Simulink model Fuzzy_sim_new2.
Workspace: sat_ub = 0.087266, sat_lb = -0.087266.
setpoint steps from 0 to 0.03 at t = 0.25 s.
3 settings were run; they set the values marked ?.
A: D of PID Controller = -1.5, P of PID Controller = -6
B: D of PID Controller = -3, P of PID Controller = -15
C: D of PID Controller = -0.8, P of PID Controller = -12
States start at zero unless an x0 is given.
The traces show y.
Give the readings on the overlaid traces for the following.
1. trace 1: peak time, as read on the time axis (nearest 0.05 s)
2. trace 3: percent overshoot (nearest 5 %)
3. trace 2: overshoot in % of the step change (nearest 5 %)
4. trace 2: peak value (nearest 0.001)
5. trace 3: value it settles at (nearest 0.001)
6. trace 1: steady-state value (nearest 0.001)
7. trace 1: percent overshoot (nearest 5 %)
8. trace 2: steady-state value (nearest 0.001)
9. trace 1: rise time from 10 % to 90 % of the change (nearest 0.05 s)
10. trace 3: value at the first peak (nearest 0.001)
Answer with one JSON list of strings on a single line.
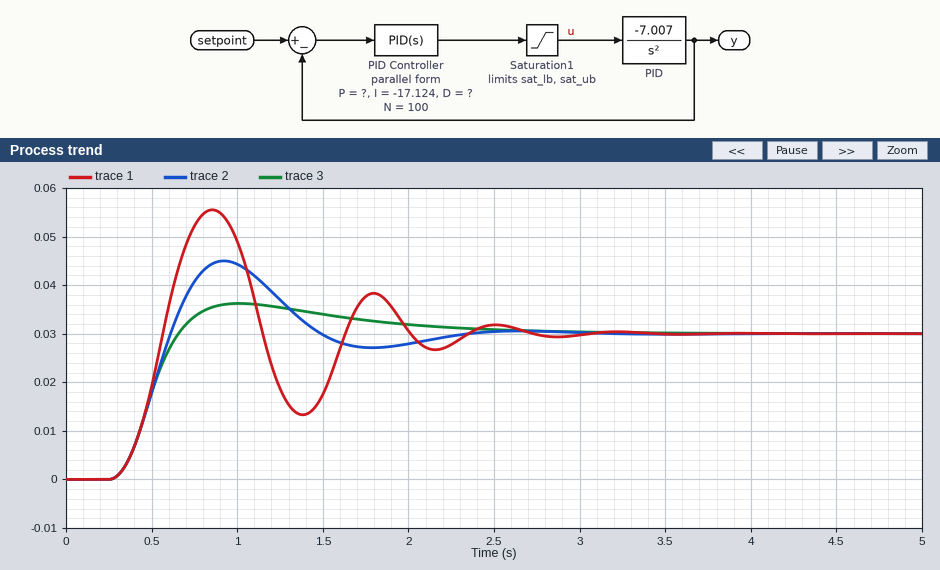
["0.85 s", "20 %", "50 %", "0.045", "0.030", "0.030", "85 %", "0.030", "0.20 s", "0.036"]
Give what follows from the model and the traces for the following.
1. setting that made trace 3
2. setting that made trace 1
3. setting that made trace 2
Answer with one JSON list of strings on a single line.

["B", "C", "A"]
